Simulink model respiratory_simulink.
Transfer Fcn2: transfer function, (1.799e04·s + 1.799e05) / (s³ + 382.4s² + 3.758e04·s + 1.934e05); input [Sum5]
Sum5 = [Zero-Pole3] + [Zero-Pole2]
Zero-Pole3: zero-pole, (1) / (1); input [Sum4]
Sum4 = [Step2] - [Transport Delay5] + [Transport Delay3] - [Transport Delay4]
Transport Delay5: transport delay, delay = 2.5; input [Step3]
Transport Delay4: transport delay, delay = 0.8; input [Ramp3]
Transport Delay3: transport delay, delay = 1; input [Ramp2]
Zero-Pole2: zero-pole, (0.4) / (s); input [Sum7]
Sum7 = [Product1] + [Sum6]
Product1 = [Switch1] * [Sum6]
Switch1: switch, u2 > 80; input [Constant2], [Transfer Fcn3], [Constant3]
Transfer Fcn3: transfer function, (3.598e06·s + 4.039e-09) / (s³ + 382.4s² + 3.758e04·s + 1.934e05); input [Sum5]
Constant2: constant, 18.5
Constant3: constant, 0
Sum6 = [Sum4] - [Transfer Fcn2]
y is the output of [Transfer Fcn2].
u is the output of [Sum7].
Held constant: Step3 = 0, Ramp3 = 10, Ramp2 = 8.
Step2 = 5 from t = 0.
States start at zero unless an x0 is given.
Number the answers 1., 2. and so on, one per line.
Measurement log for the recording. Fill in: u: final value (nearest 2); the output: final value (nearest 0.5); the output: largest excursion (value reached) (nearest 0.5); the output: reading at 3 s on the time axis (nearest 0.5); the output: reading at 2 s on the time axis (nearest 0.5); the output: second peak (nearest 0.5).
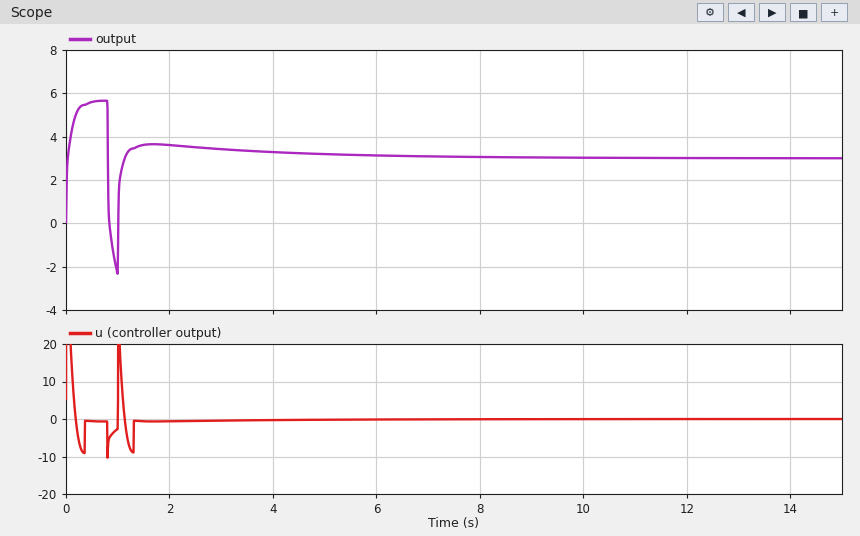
1. 0
2. 3.0
3. 5.5
4. 3.5
5. 3.5
6. 3.5
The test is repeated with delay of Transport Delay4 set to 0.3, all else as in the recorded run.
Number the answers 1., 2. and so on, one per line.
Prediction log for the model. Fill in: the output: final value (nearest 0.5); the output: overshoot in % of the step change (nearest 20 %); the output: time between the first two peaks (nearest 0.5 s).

1. 3.0
2. 80 %
3. 1.5 s
